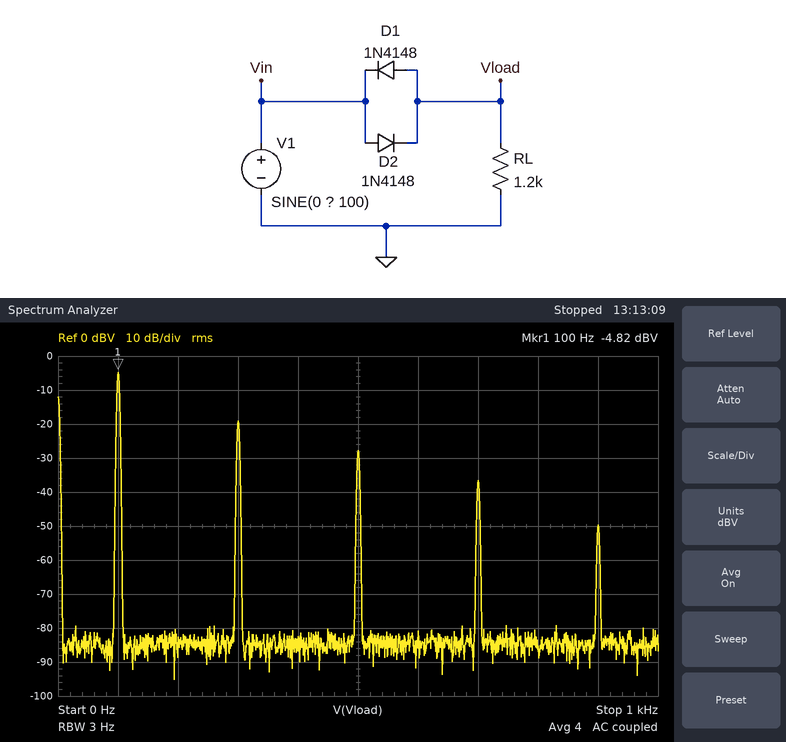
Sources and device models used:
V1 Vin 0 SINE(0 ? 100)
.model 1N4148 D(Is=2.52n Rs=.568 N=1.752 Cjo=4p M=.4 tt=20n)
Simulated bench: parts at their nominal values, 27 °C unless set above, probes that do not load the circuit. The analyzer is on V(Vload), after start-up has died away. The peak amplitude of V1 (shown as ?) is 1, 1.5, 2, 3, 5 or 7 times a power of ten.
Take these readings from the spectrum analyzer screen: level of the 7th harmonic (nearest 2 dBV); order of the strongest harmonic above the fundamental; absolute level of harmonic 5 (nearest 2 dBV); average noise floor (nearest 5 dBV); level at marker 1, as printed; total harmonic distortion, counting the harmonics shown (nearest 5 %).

-36 dBV
3
-28 dBV
-85 dBV
-4.82 dBV
20 %
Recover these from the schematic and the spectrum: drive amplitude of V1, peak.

1.5 V
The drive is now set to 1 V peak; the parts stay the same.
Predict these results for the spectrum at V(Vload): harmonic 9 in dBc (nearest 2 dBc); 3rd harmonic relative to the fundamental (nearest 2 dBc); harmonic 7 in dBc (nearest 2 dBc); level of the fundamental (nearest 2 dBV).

-38 dBc
-10 dBc
-52 dBc
-12 dBV
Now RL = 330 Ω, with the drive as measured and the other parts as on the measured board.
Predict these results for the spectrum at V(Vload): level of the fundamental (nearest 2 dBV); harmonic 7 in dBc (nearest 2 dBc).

-6 dBV
-34 dBc
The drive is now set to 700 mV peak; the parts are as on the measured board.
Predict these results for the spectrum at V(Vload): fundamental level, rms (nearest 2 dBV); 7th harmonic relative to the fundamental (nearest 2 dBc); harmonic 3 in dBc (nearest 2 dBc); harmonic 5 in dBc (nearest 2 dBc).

-20 dBV
-28 dBc
-8 dBc
-42 dBc
